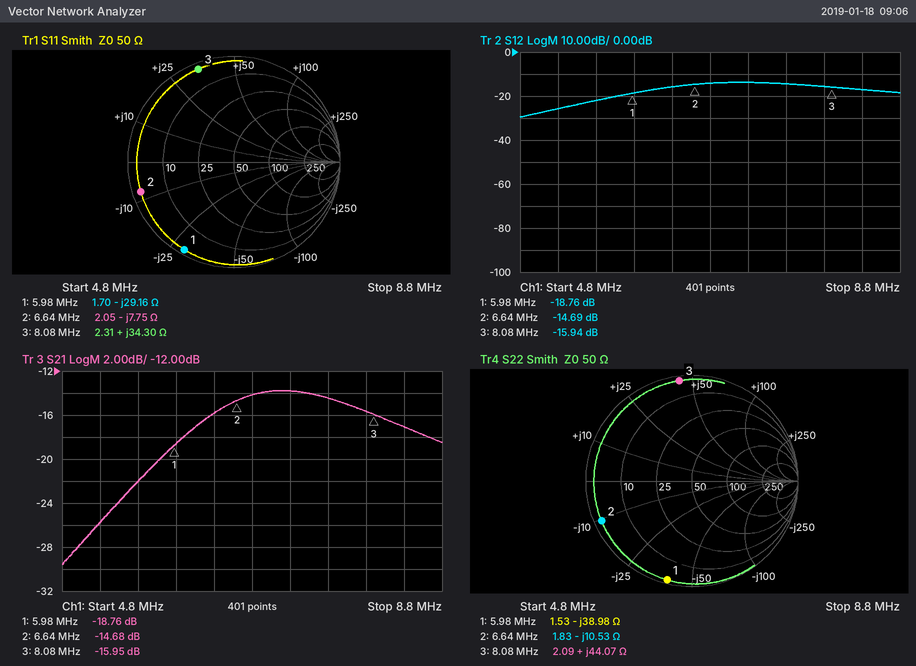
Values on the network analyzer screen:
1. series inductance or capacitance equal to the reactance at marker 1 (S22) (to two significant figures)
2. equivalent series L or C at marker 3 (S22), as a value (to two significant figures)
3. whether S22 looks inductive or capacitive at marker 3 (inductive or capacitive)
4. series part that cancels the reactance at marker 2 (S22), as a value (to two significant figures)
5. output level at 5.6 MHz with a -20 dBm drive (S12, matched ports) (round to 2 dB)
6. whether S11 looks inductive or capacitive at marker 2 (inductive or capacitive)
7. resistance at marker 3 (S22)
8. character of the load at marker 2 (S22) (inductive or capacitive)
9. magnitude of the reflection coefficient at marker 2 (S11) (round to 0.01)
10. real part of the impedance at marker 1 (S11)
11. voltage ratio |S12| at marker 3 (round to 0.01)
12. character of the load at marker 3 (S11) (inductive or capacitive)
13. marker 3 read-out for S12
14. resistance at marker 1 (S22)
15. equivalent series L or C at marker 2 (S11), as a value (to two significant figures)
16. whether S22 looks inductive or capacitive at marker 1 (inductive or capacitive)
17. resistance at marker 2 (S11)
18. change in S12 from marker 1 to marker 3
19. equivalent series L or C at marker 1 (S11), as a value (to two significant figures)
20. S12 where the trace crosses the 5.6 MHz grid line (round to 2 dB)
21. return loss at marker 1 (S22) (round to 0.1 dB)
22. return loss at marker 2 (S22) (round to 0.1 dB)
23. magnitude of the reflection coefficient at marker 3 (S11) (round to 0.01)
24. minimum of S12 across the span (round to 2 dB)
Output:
680 pF
870 nH
inductive
250 nH
-42 dBm
capacitive
2.09 Ω
capacitive
0.92
1.70 Ω
0.16
inductive
-15.94 dB
1.53 Ω
3.1 nF
capacitive
2.05 Ω
2.82 dB
910 pF
-22 dB
0.3 dB
0.6 dB
0.94
-30 dB
